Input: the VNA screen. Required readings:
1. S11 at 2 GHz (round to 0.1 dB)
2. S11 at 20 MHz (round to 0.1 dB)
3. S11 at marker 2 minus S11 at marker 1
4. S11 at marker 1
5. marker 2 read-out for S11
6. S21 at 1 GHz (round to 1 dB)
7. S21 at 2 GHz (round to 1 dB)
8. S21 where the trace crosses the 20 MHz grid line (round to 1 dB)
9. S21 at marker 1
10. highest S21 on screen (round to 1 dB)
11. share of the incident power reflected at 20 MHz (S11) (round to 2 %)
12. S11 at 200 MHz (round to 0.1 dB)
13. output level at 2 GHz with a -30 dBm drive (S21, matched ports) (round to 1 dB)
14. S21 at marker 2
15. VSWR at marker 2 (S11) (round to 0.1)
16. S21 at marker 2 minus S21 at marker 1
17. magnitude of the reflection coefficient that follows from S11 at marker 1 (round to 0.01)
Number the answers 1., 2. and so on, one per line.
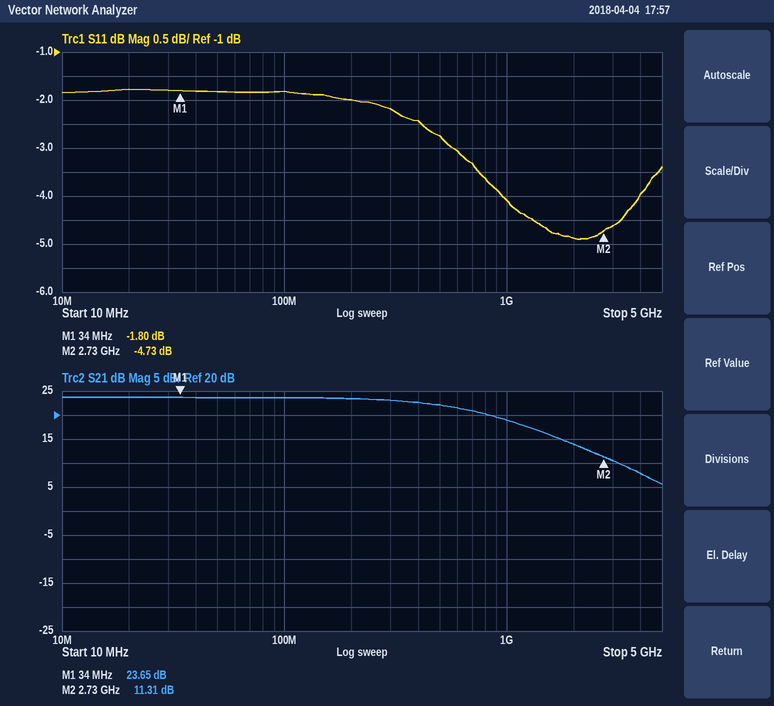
1. -4.9 dB
2. -1.8 dB
3. -2.93 dB
4. -1.80 dB
5. -4.73 dB
6. 19 dB
7. 14 dB
8. 24 dB
9. 23.65 dB
10. 24 dB
11. 66 %
12. -2.0 dB
13. -16 dBm
14. 11.31 dB
15. 3.8
16. -12.34 dB
17. 0.81
